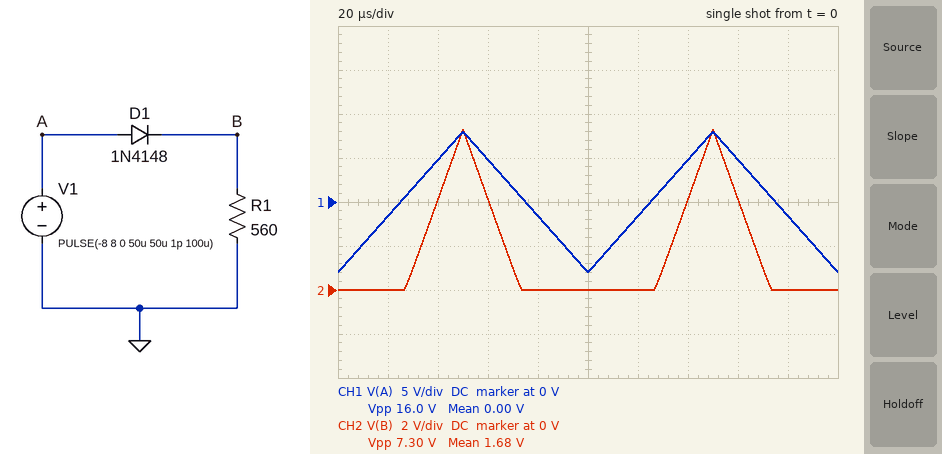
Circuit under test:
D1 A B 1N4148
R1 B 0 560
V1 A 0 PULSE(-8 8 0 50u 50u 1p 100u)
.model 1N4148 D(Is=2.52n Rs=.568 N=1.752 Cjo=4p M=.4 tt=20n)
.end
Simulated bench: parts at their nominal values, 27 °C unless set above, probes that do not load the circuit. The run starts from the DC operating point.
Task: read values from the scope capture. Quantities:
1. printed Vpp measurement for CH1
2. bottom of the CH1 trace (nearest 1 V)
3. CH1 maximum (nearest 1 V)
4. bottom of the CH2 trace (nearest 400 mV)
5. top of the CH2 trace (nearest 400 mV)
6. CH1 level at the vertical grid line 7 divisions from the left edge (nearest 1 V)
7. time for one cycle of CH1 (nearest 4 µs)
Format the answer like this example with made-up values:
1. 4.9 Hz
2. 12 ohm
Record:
1. 16.0 V
2. -8 V
3. 8 V
4. 0 V
5. 7.2 V
6. 5 V
7. 100 µs
